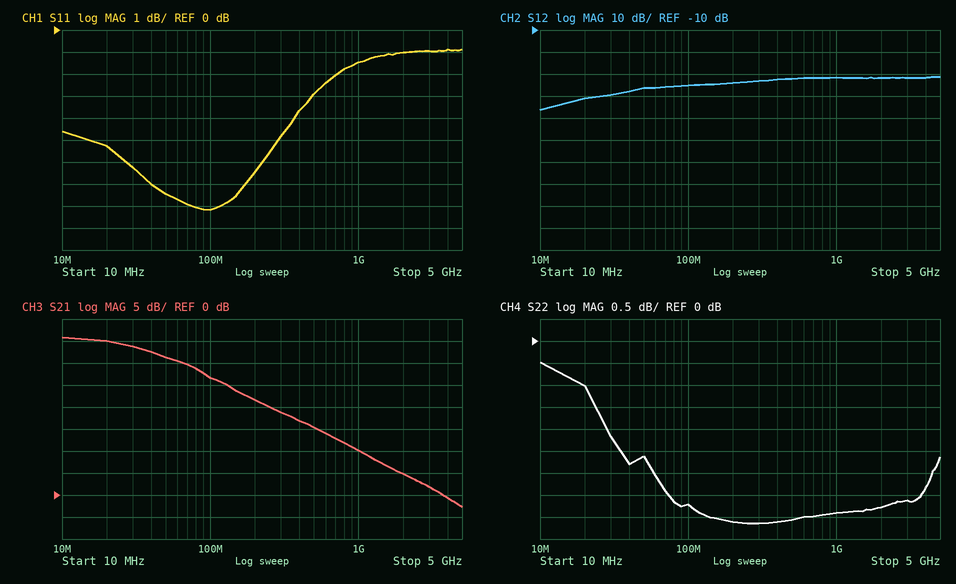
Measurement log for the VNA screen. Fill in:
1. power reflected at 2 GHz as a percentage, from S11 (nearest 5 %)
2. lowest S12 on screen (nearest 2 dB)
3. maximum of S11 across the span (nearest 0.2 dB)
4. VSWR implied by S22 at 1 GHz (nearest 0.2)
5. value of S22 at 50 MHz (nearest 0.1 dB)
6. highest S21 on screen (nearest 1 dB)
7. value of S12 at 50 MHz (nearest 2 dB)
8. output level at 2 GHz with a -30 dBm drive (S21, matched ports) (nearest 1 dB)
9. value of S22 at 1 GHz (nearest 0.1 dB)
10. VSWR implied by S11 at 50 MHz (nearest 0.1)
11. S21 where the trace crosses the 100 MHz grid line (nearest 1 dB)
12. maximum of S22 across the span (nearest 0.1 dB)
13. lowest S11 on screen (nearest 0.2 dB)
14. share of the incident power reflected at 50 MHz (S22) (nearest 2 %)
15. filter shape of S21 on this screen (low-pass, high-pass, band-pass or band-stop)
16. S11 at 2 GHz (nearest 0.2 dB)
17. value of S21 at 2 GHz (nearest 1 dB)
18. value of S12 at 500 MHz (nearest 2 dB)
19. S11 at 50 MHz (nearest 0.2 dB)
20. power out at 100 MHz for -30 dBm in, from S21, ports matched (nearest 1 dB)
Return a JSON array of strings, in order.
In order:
["80 %", "-46 dB", "-0.8 dB", "4.6", "-2.6 dB", "36 dB", "-36 dB", "-25 dBm", "-3.9 dB", "2.5", "27 dB", "-0.5 dB", "-8.2 dB", "54 %", "low-pass", "-1.0 dB", "5 dB", "-32 dB", "-7.4 dB", "-3 dBm"]
